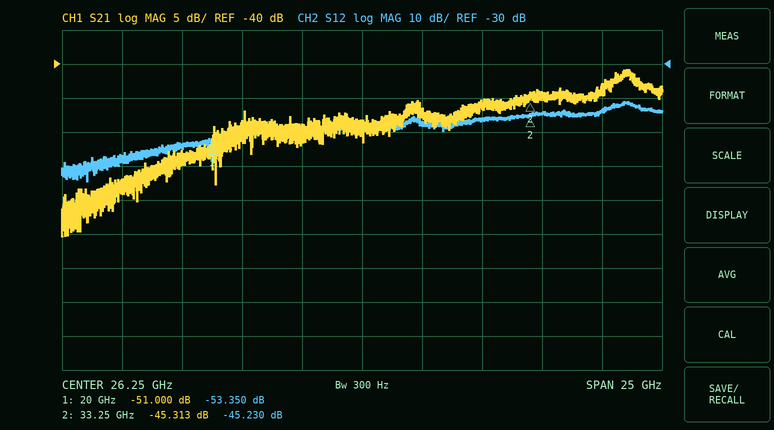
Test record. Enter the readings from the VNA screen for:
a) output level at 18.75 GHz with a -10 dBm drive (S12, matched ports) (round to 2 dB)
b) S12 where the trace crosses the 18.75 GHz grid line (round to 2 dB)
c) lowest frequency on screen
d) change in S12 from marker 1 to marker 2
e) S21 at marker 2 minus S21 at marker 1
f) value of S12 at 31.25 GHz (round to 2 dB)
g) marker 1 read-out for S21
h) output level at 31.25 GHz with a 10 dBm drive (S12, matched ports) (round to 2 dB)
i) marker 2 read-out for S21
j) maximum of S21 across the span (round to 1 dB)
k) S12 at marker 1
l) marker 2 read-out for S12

-64 dBm
-54 dB
13.75 GHz
8.120 dB
5.687 dB
-46 dB
-51.000 dB
-36 dBm
-45.313 dB
-41 dB
-53.350 dB
-45.230 dB
